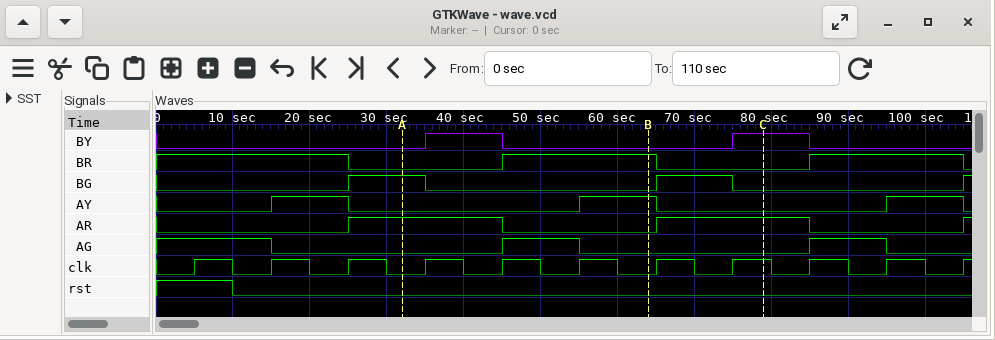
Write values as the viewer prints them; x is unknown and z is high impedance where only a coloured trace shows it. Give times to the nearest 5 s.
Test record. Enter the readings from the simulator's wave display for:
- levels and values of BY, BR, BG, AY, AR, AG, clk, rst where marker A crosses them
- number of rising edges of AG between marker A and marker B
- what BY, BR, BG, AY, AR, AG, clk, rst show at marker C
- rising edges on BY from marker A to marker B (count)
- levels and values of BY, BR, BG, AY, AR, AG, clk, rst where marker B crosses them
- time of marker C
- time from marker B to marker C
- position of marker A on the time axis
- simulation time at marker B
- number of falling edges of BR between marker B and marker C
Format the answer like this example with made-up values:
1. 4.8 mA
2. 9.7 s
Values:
1. BY=0, BR=0, BG=1, AY=0, AR=1, AG=0, clk=0, rst=0
2. 1
3. BY=1, BR=0, BG=0, AY=0, AR=1, AG=0, clk=1, rst=0
4. 1
5. BY=0, BR=1, BG=0, AY=1, AR=0, AG=0, clk=0, rst=0
6. 80 s
7. 15 s
8. 30 s
9. 65 s
10. 1
